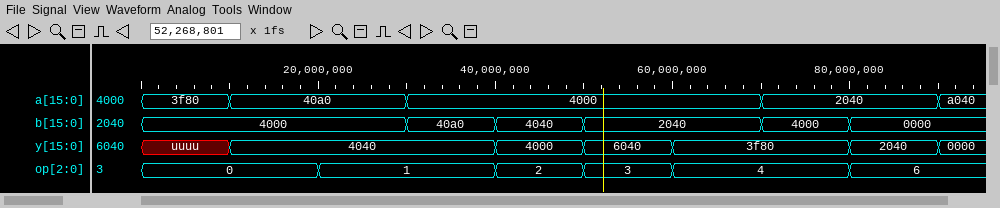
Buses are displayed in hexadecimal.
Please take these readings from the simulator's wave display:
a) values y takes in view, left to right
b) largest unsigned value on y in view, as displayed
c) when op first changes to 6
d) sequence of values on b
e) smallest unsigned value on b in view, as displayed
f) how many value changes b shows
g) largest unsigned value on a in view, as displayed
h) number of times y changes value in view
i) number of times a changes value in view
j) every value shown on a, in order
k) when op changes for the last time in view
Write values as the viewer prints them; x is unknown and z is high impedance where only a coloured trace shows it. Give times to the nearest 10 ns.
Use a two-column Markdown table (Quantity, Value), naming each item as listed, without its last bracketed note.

| Quantity | Value |
|---|---|
| values y takes in view, left to right | uuuu, 4040, 4000, 6040, 3f80, 2040, 0000 |
| largest unsigned value on y in view, as displayed | 6040 |
| when op first changes to 6 | 80 ns |
| sequence of values on b | 4000, 40a0, 4040, 2040, 4000, 0000 |
| smallest unsigned value on b in view, as displayed | 0000 |
| how many value changes b shows | 5 |
| largest unsigned value on a in view, as displayed | a040 |
| number of times y changes value in view | 6 |
| number of times a changes value in view | 4 |
| every value shown on a, in order | 3f80, 40a0, 4000, 2040, a040 |
| when op changes for the last time in view | 80 ns |
